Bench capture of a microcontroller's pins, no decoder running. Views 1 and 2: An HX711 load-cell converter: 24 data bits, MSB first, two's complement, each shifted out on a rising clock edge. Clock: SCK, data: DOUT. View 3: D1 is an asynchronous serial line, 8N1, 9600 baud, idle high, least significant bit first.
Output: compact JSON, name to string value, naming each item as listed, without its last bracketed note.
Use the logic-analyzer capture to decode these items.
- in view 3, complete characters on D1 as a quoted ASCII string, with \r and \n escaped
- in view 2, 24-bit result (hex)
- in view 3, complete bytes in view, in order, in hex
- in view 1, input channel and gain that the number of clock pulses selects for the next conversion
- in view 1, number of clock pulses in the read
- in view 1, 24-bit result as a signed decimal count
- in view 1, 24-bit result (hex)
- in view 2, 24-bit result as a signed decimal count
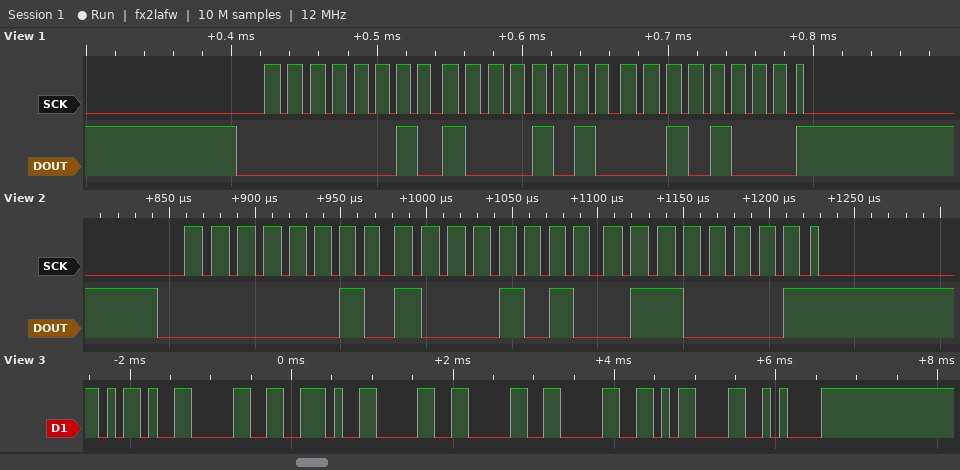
{"in view 3, complete characters on D1 as a quoted ASCII string, with \\r and \\n escaped": "\"-0.000\\r\\n\"", "in view 2, 24-bit result": "0x028A61", "in view 3, complete bytes in view, in order, in hex": "2D 30 2E 30 30 30 0D 0A", "in view 1, input channel and gain that the number of clock pulses selects for the next conversion": "channel A, gain 128", "in view 1, number of clock pulses in the read": "25", "in view 1, 24-bit result as a signed decimal count": "166440", "in view 1, 24-bit result": "0x028A28", "in view 2, 24-bit result as a signed decimal count": "166497"}
